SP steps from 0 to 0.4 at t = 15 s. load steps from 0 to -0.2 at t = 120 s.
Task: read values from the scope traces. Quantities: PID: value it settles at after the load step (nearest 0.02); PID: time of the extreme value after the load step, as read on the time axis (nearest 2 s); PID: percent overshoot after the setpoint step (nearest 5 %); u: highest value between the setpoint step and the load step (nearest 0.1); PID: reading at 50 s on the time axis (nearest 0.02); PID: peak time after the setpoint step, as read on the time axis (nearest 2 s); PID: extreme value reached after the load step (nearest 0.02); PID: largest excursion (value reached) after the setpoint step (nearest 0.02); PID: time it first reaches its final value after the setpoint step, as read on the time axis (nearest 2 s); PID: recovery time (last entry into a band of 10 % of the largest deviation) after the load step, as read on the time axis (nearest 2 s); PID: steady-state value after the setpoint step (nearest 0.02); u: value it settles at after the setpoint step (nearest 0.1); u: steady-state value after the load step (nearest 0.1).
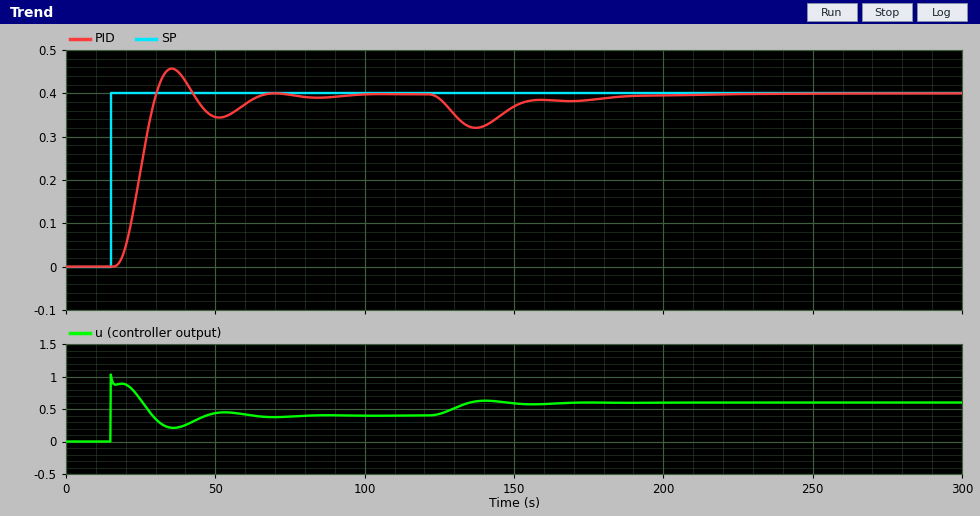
0.40
138 s
15 %
1.0
0.34
36 s
0.32
0.46
30 s
186 s
0.40
0.4
0.6
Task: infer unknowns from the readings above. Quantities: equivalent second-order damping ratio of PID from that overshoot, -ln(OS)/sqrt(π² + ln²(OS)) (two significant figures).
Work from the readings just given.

0.52
